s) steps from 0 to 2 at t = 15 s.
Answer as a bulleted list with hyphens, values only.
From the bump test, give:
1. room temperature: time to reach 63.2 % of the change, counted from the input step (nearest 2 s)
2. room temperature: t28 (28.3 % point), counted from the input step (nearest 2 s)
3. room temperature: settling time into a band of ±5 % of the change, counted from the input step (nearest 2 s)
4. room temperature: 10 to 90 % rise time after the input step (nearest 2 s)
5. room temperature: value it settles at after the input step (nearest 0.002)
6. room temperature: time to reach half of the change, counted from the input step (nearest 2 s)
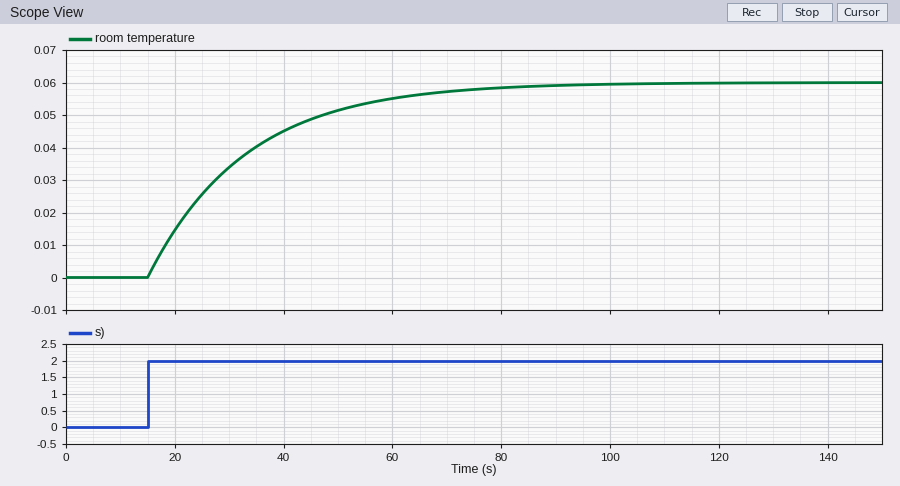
- 18 s
- 6 s
- 54 s
- 40 s
- 0.060
- 12 s
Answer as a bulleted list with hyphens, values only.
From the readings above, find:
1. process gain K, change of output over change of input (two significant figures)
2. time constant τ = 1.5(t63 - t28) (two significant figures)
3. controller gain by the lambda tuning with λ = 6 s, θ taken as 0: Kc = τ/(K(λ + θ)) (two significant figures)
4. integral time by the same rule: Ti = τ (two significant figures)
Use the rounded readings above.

- 0.030
- 18 s
- 100
- 18 s
